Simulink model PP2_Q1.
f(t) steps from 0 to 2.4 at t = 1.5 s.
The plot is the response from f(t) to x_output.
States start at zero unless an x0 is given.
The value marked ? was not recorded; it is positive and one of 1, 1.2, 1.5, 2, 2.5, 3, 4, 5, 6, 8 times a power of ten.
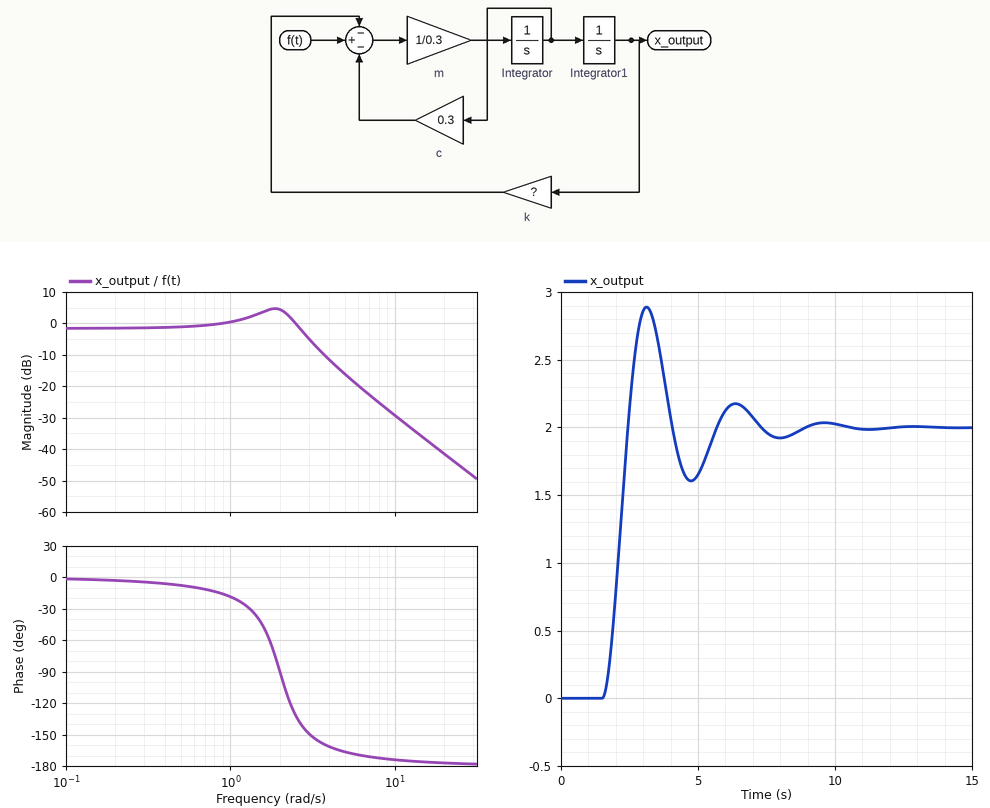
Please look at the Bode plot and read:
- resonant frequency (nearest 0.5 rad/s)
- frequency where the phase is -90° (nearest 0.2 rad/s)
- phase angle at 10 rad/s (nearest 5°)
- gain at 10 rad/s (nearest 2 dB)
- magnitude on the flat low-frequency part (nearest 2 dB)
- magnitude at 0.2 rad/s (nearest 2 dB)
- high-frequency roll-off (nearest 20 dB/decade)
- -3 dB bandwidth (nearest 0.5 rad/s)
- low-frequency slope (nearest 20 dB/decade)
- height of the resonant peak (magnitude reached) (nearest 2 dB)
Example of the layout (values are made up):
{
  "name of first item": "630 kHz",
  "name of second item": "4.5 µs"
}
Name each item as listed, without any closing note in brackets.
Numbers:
{
  "resonant frequency": "2.0 rad/s",
  "frequency where the phase is -90°": "2.0 rad/s",
  "phase angle at 10 rad/s": "-175°",
  "gain at 10 rad/s": "-30 dB",
  "magnitude on the flat low-frequency part": "-2 dB",
  "magnitude at 0.2 rad/s": "-2 dB",
  "high-frequency roll-off": "-40 dB/decade",
  "-3 dB bandwidth": "3.0 rad/s",
  "low-frequency slope": "0 dB/decade",
  "height of the resonant peak (magnitude reached)": "4 dB"
}
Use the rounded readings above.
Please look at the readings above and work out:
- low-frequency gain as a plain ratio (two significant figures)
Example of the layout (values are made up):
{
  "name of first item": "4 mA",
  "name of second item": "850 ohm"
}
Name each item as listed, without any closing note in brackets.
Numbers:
{
  "low-frequency gain as a plain ratio": "0.79"
}
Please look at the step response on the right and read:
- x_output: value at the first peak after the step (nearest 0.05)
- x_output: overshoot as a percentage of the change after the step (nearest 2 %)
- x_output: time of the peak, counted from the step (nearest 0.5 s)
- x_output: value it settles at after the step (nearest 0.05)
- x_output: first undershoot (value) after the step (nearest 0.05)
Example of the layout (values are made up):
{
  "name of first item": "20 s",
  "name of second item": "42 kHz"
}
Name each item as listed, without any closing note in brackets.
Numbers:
{
  "x_output: value at the first peak after the step": "2.90",
  "x_output: overshoot as a percentage of the change after the step": "44 %",
  "x_output: time of the peak, counted from the step": "1.5 s",
  "x_output: value it settles at after the step": "2.00",
  "x_output: first undershoot (value) after the step": "1.60"
}
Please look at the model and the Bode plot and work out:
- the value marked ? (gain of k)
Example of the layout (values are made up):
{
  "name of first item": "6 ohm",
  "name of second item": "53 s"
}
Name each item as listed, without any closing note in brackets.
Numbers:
{
  "the value marked ?": "1.2"
}
